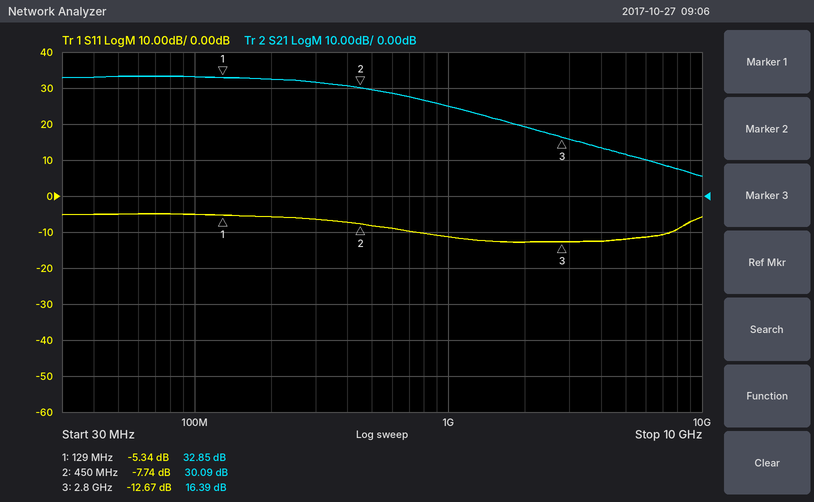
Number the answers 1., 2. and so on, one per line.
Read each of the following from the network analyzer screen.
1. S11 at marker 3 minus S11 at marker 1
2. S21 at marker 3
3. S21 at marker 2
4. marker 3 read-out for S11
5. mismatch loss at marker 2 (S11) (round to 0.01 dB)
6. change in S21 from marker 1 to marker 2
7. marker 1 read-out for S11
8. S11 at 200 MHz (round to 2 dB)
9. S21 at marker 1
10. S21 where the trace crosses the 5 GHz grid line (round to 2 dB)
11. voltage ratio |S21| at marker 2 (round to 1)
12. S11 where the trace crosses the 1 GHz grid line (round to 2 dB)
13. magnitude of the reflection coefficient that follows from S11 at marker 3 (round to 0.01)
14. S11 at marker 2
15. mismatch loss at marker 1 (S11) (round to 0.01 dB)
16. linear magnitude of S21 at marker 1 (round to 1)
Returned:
1. -7.33 dB
2. 16.39 dB
3. 30.09 dB
4. -12.67 dB
5. 0.80 dB
6. -2.76 dB
7. -5.34 dB
8. -6 dB
9. 32.85 dB
10. 12 dB
11. 32
12. -12 dB
13. 0.23
14. -7.74 dB
15. 1.50 dB
16. 44
